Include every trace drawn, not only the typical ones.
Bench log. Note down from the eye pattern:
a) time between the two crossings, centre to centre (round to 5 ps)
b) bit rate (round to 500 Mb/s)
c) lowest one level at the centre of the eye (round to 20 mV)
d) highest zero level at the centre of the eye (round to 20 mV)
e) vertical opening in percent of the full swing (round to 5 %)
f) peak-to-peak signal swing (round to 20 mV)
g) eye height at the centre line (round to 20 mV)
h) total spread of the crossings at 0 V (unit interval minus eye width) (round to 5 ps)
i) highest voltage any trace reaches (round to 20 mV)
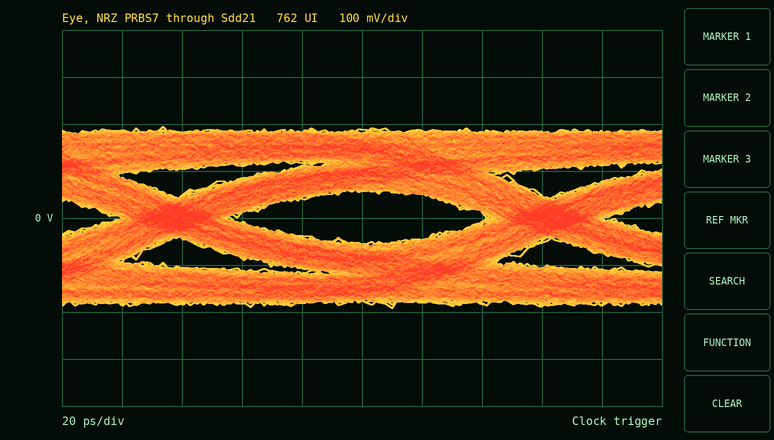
125 ps
8.0 Gb/s
60 mV
-60 mV
30 %
380 mV
120 mV
40 ps
200 mV
